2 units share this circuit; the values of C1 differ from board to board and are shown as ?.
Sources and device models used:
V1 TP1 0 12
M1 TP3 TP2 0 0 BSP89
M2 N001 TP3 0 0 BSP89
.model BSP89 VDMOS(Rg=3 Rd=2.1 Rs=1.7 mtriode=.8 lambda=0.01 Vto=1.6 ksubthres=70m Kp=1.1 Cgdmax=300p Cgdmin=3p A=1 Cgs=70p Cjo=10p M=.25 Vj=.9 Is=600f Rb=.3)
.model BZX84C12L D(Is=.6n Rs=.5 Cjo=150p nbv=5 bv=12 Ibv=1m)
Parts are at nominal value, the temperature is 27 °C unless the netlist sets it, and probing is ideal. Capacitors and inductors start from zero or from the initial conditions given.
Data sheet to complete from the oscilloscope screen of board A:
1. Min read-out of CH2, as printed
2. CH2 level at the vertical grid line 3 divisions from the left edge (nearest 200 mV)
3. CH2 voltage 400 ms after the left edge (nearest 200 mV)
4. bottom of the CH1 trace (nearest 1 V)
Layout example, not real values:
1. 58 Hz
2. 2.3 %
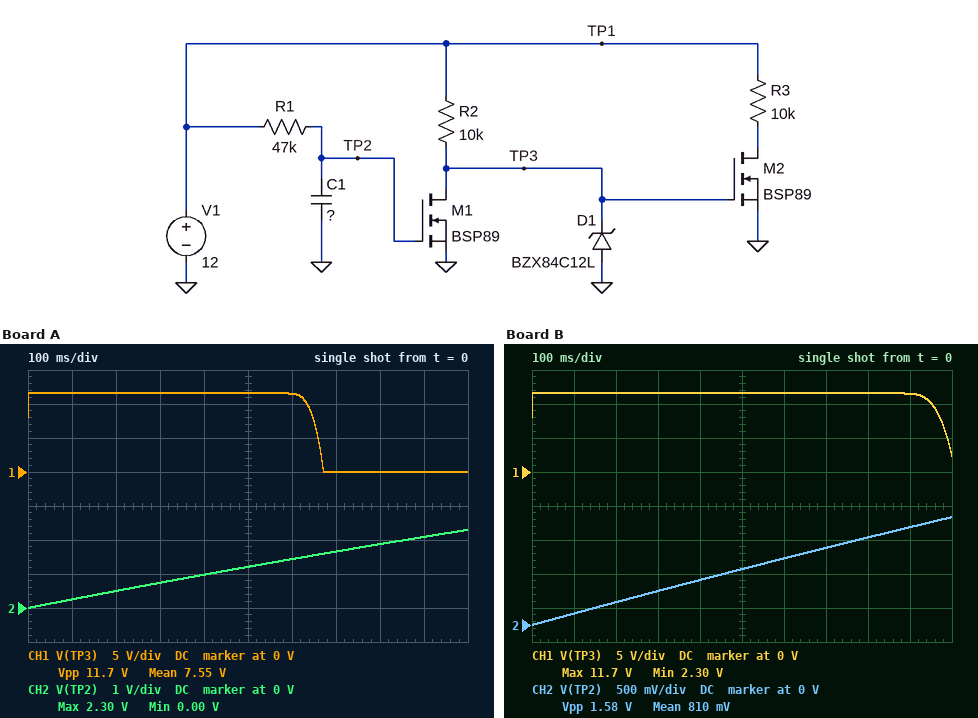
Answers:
1. 0.00 V
2. 800 mV
3. 1.0 V
4. 0 V
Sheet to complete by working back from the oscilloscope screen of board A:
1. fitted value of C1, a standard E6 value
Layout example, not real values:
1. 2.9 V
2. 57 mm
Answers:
1. 100 µF
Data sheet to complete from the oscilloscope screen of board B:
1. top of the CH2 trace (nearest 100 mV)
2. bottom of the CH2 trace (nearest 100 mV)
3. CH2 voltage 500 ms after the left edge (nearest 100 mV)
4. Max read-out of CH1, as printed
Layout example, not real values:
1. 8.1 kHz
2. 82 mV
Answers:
1. 1.6 V
2. 0 V
3. 800 mV
4. 11.7 V
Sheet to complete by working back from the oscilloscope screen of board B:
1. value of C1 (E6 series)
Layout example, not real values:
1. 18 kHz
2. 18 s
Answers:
1. 150 µF
